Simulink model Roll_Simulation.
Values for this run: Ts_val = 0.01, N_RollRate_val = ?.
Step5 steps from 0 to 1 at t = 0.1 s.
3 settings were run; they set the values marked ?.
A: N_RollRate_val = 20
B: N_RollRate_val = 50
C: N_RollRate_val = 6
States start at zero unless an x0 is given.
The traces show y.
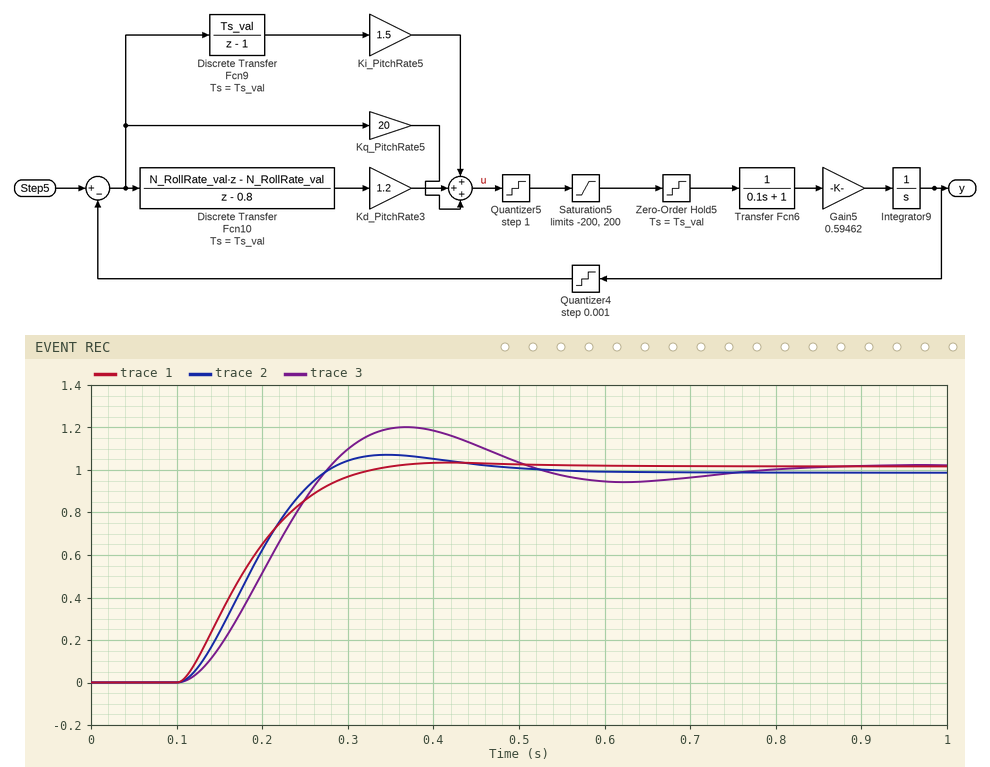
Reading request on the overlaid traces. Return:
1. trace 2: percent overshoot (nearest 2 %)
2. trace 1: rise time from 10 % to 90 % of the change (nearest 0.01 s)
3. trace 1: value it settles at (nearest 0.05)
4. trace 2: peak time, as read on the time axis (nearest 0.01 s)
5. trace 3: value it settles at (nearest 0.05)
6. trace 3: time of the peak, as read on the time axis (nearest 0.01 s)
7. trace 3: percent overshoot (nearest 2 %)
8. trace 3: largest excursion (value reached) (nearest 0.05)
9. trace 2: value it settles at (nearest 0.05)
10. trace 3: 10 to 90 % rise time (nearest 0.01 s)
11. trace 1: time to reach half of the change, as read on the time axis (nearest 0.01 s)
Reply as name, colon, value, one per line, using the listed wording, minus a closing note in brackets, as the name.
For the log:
trace 2: percent overshoot: 8 %
trace 1: rise time from 10 % to 90 % of the change: 0.15 s
trace 1: value it settles at: 1.00
trace 2: peak time, as read on the time axis: 0.35 s
trace 3: value it settles at: 1.00
trace 3: time of the peak, as read on the time axis: 0.37 s
trace 3: percent overshoot: 18 %
trace 3: largest excursion (value reached): 1.20
trace 2: value it settles at: 1.00
trace 3: 10 to 90 % rise time: 0.12 s
trace 1: time to reach half of the change, as read on the time axis: 0.18 s
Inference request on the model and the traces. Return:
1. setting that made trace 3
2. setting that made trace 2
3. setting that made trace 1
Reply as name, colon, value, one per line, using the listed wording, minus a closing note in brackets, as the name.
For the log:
setting that made trace 3: C
setting that made trace 2: A
setting that made trace 1: B
